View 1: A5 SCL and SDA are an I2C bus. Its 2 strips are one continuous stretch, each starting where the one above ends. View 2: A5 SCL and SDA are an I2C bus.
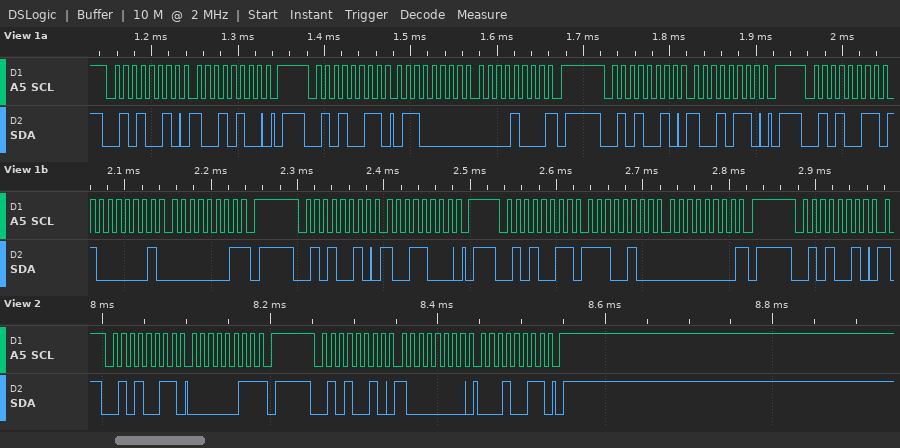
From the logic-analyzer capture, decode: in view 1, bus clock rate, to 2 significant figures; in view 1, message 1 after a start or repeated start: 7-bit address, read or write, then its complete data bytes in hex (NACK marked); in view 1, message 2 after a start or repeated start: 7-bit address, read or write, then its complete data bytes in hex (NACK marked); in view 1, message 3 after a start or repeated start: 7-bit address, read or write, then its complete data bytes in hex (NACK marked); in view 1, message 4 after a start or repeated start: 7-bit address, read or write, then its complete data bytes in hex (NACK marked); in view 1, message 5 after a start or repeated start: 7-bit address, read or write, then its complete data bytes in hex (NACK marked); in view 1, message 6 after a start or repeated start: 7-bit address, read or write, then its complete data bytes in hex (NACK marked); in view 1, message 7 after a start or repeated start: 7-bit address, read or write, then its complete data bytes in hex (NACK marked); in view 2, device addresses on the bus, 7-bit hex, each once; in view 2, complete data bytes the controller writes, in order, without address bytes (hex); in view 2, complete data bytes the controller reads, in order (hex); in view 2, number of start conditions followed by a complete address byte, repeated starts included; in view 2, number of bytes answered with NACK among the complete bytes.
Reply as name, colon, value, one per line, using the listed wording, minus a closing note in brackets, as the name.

in view 1, bus clock rate, to 2 significant figures: 100 kHz
in view 1, message 1 after a start or repeated start: 7-bit address, read or write, then its complete data bytes in hex: 0x29 write: 94
in view 1, message 2 after a start or repeated start: 7-bit address, read or write, then its complete data bytes in hex: 0x29 read: 60 08 NACK
in view 1, message 3 after a start or repeated start: 7-bit address, read or write, then its complete data bytes in hex: 0x29 write: 96
in view 1, message 4 after a start or repeated start: 7-bit address, read or write, then its complete data bytes in hex: 0x29 read: 81 01 NACK
in view 1, message 5 after a start or repeated start: 7-bit address, read or write, then its complete data bytes in hex: 0x29 write: 98
in view 1, message 6 after a start or repeated start: 7-bit address, read or write, then its complete data bytes in hex: 0x29 read: E4 00 NACK
in view 1, message 7 after a start or repeated start: 7-bit address, read or write, then its complete data bytes in hex: 0x29 write
in view 2, device addresses on the bus, 7-bit hex, each once: 0x29
in view 2, complete data bytes the controller writes, in order, without address bytes: 80 13
in view 2, complete data bytes the controller reads, in order: 03
in view 2, number of start conditions followed by a complete address byte, repeated starts included: 2
in view 2, number of bytes answered with NACK among the complete bytes: 1
